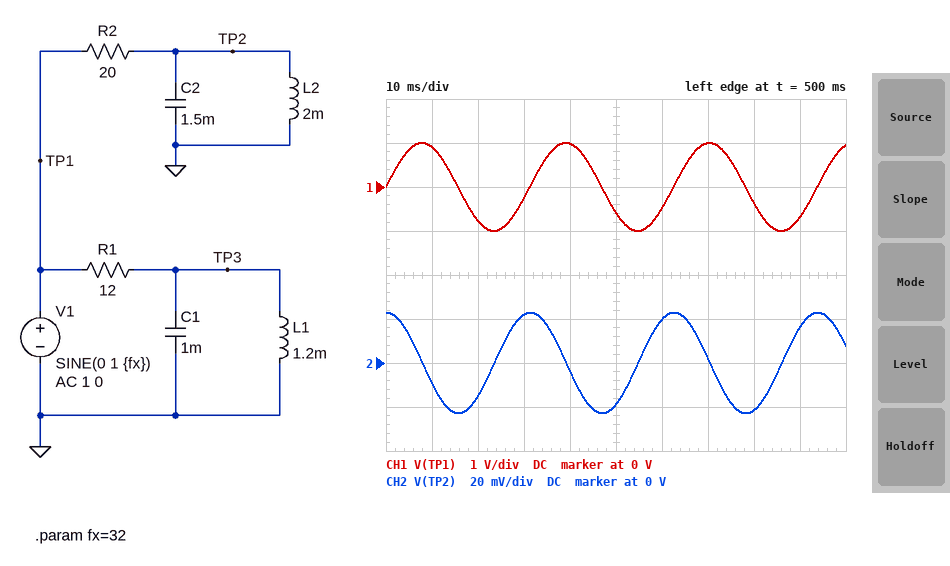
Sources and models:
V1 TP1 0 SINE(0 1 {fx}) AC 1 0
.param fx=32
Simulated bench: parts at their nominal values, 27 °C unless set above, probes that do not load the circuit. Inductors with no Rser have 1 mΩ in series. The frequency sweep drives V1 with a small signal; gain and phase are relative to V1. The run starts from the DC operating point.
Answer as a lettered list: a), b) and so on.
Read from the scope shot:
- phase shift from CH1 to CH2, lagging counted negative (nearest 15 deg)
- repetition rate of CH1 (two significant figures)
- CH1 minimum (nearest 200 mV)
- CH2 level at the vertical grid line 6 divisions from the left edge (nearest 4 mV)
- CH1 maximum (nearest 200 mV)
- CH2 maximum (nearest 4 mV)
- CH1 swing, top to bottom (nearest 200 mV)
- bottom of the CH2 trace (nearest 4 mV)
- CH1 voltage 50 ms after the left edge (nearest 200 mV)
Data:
a) 90 deg
b) 32 Hz
c) -1.0 V
d) 20 mV
e) 1.0 V
f) 24 mV
g) 2.0 V
h) -24 mV
i) -600 mV
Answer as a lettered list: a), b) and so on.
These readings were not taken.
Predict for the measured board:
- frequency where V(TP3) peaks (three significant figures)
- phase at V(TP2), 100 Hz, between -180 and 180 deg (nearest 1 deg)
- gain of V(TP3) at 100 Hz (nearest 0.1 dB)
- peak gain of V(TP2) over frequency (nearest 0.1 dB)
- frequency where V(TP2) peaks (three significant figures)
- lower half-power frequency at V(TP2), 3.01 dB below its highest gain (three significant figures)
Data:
a) 145 Hz
b) -71 deg
c) -18.5 dB
d) -0.1 dB
e) 91.9 Hz
f) 89.2 Hz
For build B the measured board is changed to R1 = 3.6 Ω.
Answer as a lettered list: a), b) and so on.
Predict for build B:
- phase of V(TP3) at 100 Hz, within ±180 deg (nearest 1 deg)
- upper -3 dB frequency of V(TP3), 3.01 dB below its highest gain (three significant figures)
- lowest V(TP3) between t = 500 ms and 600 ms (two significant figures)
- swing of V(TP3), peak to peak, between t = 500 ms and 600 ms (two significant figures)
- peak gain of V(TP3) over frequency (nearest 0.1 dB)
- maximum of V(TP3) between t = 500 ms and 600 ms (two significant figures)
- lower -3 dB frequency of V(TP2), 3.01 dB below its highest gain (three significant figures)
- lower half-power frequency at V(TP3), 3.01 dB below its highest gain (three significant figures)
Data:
a) 68 deg
b) 169 Hz
c) -70 mV
d) 140 mV
e) 0 dB
f) 70 mV
g) 89.2 Hz
h) 125 Hz
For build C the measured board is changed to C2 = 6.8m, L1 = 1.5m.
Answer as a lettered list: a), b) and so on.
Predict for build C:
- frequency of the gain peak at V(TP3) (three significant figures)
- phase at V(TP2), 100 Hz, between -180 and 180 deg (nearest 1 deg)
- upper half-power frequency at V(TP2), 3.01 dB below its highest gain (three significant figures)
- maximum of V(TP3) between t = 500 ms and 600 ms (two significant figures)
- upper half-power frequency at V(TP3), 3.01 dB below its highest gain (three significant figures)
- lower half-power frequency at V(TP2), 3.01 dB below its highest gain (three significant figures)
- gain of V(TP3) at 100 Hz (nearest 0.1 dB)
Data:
a) 130 Hz
b) -89 deg
c) 43.8 Hz
d) 27 mV
e) 137 Hz
f) 42.5 Hz
g) -14.5 dB
